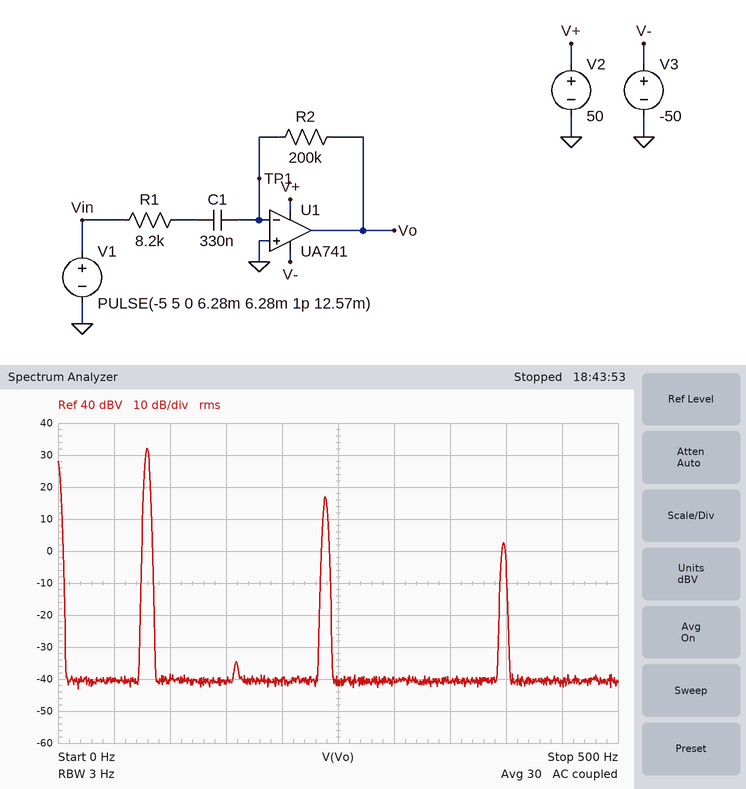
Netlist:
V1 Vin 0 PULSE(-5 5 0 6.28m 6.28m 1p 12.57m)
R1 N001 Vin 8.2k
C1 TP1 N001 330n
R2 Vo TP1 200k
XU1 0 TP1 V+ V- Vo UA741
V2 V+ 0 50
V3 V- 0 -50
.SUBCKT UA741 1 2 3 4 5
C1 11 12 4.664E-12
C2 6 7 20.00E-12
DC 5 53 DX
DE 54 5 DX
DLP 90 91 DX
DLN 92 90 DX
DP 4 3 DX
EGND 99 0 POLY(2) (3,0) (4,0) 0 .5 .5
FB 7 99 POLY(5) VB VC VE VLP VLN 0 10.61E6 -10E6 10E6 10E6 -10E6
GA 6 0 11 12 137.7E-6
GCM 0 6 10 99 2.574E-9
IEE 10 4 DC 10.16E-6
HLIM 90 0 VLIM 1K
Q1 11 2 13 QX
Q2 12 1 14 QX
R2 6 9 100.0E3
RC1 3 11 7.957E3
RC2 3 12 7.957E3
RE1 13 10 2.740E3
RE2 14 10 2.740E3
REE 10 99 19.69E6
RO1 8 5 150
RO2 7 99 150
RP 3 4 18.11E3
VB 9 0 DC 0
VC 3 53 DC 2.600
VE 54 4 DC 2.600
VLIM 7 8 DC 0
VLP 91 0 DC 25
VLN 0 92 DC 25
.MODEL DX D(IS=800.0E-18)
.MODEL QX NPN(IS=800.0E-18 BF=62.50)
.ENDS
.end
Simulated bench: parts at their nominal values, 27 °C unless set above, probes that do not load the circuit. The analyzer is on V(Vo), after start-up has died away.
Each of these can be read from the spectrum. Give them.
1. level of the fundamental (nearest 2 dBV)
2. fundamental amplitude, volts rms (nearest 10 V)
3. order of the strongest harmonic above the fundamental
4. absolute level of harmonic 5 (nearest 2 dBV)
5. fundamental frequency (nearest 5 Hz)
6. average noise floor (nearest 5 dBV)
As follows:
32 dBV
40 V
3
2 dBV
80 Hz
-40 dBV
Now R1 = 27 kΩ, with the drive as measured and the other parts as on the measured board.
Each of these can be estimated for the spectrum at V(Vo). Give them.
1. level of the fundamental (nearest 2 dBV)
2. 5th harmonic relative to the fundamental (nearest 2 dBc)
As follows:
26 dBV
-28 dBc
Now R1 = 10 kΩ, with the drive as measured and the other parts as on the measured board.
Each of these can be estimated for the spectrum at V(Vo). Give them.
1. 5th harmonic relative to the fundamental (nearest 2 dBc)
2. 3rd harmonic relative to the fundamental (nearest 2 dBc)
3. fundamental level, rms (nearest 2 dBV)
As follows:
-26 dBc
-18 dBc
32 dBV
